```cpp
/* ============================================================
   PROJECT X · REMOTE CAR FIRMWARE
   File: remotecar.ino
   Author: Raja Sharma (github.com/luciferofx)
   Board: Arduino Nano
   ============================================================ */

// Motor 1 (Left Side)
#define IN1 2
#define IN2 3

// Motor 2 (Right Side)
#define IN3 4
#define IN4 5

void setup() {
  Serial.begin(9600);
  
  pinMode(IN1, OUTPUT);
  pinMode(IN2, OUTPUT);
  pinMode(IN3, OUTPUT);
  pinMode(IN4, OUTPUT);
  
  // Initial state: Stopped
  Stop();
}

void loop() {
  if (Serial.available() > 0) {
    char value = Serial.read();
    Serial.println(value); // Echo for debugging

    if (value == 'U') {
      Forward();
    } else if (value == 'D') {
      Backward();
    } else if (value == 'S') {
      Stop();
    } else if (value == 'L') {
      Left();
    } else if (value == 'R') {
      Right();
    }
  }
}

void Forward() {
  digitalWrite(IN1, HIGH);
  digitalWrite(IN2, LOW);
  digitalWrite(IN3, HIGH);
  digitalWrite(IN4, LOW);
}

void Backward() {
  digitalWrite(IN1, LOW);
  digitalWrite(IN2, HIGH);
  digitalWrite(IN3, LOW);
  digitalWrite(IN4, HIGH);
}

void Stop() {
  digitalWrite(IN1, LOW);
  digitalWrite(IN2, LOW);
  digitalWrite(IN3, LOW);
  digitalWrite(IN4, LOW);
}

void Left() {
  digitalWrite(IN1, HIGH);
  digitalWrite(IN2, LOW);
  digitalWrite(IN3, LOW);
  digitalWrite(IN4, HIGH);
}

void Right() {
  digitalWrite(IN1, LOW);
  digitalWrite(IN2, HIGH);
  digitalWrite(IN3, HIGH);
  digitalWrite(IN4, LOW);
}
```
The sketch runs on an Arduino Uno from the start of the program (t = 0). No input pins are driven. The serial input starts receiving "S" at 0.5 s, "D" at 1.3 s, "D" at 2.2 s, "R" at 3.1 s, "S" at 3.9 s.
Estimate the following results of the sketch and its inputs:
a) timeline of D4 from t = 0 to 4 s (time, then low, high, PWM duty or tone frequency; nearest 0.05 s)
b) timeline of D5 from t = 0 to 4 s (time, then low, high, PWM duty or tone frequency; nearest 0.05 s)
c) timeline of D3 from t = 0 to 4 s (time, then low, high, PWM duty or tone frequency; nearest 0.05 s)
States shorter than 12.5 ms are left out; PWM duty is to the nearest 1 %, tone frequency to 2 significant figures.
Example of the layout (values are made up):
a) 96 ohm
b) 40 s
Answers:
a) 0 s low; 3.1 s high; 3.9 s low
b) 0 s low; 1.3 s high; 3.1 s low
c) 0 s low; 1.3 s high; 3.9 s low
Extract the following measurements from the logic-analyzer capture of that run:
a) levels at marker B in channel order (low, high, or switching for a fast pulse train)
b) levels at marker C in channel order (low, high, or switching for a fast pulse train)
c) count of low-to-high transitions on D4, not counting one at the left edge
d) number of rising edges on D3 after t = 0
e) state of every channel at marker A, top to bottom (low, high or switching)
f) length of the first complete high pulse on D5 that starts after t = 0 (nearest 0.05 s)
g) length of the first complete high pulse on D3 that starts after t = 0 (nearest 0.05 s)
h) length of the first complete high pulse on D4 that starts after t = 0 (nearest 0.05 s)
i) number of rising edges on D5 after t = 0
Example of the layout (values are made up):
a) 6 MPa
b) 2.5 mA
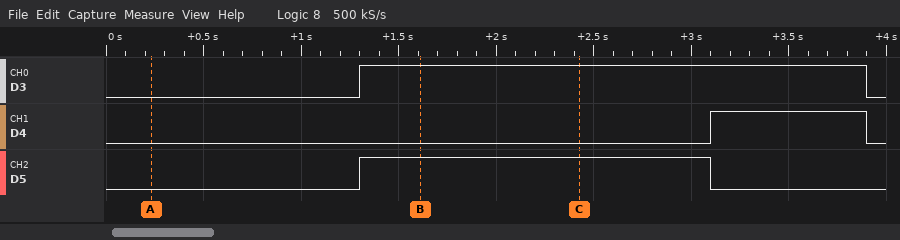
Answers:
a) D3 high, D4 low, D5 high
b) D3 high, D4 low, D5 high
c) 1
d) 1
e) D3 low, D4 low, D5 low
f) 1.80 s
g) 2.60 s
h) 0.80 s
i) 1
